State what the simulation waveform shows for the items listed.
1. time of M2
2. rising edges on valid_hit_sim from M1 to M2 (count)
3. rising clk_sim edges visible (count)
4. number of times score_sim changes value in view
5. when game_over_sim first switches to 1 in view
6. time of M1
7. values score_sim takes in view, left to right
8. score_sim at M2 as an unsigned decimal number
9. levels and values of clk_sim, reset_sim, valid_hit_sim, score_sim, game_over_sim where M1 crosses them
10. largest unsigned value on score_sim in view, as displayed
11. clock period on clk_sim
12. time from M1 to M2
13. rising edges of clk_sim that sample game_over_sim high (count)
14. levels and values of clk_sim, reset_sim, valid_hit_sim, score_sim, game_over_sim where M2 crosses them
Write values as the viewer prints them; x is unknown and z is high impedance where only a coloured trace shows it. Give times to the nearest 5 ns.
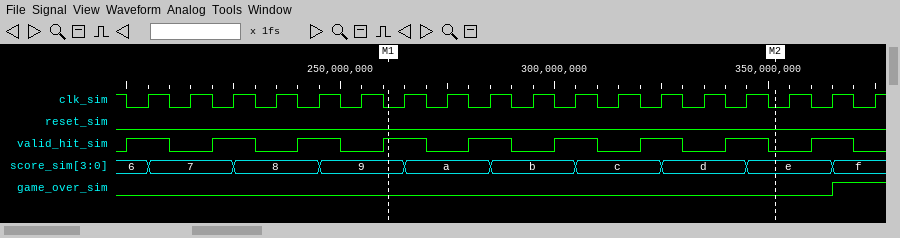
350 ns
4
18
9
365 ns
260 ns
6, 7, 8, 9, a, b, c, d, e, f
14
clk_sim=0, reset_sim=0, valid_hit_sim=1, score_sim=9, game_over_sim=0
f
10 ns
90 ns
1
clk_sim=0, reset_sim=0, valid_hit_sim=0, score_sim=e, game_over_sim=0
